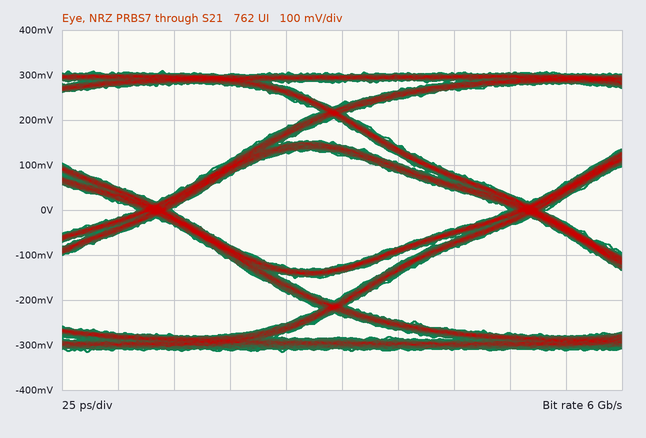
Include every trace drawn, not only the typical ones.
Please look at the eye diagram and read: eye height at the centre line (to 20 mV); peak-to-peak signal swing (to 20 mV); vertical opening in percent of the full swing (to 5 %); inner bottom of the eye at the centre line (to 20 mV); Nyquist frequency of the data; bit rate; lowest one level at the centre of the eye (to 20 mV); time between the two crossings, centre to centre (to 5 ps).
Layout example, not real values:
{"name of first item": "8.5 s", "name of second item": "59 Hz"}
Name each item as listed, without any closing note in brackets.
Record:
{"eye height at the centre line": "240 mV", "peak-to-peak signal swing": "620 mV", "vertical opening in percent of the full swing": "40 %", "inner bottom of the eye at the centre line": "-120 mV", "Nyquist frequency of the data": "3 GHz", "bit rate": "6 Gb/s", "lowest one level at the centre of the eye": "120 mV", "time between the two crossings, centre to centre": "165 ps"}
